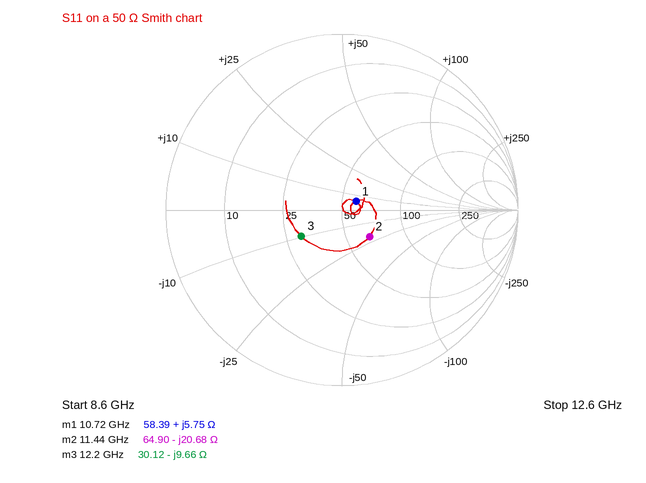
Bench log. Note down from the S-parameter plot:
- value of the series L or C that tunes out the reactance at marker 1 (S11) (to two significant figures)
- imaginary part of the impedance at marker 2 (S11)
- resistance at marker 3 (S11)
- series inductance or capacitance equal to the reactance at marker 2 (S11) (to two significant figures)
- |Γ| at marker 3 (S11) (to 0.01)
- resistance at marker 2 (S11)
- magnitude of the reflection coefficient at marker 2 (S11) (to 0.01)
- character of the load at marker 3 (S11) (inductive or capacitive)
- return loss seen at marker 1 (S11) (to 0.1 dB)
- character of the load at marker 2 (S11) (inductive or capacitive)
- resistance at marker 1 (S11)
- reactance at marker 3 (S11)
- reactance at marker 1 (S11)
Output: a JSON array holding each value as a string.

["2.6 pF", "-20.68 Ω", "30.12 Ω", "670 fF", "0.27", "64.90 Ω", "0.22", "capacitive", "20.6 dB", "capacitive", "58.39 Ω", "-9.66 Ω", "+5.75 Ω"]
